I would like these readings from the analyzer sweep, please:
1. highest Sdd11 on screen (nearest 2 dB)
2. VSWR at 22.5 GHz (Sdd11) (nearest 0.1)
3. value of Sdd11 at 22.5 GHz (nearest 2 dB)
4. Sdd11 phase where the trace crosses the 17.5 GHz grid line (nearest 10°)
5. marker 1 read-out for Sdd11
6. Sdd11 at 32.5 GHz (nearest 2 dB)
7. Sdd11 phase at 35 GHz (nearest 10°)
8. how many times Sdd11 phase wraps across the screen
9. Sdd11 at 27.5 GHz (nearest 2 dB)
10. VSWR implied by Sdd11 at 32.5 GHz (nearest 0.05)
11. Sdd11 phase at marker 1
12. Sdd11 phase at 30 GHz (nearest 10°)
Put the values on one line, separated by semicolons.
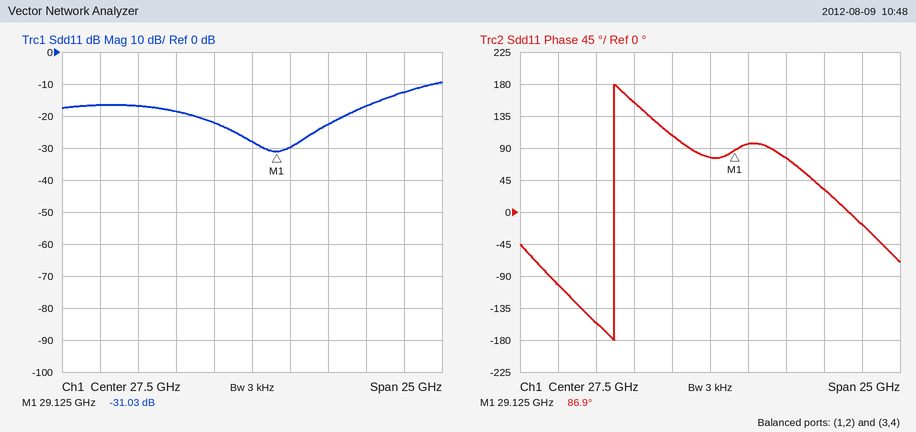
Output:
-10 dB; 1.3; -18 dB; -100°; -31.03 dB; -22 dB; 30°; 1; -28 dB; 1.15; 86.9°; 100°
